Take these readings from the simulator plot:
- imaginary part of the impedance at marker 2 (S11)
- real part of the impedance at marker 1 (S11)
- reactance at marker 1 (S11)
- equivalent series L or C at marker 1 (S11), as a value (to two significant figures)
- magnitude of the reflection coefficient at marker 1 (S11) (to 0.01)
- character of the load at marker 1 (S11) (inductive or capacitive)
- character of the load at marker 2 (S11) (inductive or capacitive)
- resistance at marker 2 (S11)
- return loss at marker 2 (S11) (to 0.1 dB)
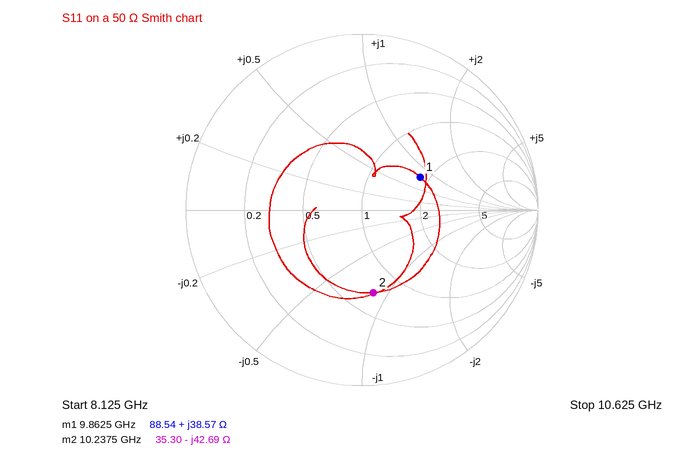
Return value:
-42.69 Ω
88.54 Ω
+38.57 Ω
620 pH
0.38
inductive
capacitive
35.30 Ω
6.5 dB
